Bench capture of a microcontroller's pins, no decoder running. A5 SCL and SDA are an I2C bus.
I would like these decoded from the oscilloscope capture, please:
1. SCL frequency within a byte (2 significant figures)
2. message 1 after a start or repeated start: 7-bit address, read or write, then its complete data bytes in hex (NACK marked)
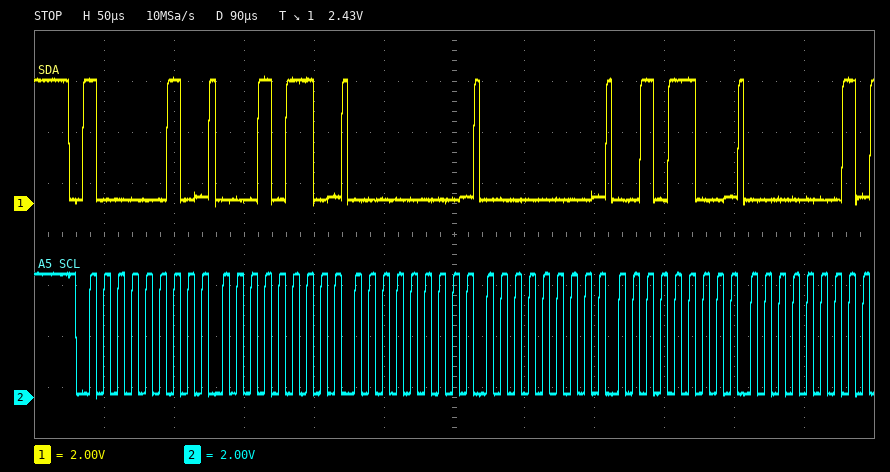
100 kHz
0x41 write: 16 00 00 2C 01
